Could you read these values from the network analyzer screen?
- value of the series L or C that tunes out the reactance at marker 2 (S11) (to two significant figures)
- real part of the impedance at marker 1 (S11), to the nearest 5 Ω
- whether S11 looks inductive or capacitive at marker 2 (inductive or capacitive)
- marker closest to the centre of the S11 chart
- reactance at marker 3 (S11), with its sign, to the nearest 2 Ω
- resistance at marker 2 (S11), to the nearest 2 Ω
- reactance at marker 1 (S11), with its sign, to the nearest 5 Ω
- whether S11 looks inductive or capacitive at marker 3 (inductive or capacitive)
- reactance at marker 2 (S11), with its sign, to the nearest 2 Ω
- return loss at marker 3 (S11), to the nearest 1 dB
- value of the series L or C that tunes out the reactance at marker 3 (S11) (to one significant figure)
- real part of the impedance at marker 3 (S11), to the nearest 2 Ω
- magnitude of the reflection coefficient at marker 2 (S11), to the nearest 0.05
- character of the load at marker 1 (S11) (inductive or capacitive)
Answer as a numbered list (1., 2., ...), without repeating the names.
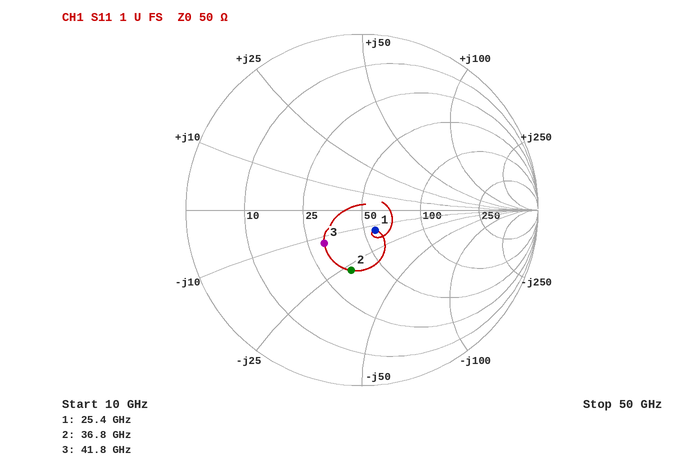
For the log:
1. 120 pH
2. 55 Ω
3. capacitive
4. marker 1
5. -12 Ω
6. 36 Ω
7. -15 Ω
8. capacitive
9. -28 Ω
10. 11 dB
11. 50 pH
12. 30 Ω
13. 0.35
14. capacitive
